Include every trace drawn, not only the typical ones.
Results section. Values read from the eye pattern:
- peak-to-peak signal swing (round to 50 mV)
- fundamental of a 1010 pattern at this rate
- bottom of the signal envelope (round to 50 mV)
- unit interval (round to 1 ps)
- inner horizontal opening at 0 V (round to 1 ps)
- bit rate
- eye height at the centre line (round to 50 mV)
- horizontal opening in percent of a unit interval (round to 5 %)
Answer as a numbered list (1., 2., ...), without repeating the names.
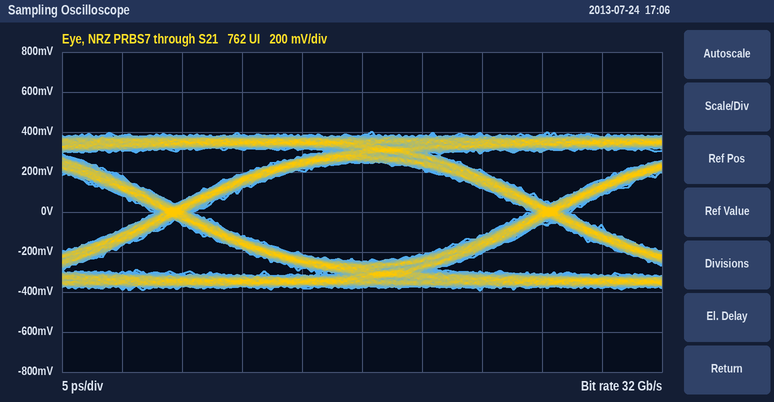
1. 800 mV
2. 16 GHz
3. -400 mV
4. 31 ps
5. 28 ps
6. 32 Gb/s
7. 500 mV
8. 90 %
